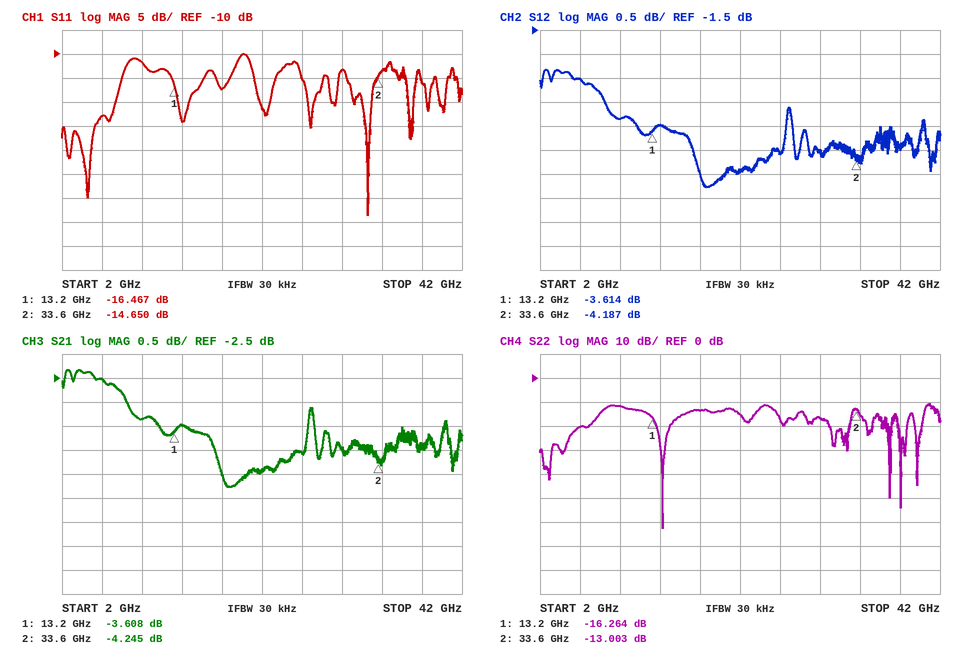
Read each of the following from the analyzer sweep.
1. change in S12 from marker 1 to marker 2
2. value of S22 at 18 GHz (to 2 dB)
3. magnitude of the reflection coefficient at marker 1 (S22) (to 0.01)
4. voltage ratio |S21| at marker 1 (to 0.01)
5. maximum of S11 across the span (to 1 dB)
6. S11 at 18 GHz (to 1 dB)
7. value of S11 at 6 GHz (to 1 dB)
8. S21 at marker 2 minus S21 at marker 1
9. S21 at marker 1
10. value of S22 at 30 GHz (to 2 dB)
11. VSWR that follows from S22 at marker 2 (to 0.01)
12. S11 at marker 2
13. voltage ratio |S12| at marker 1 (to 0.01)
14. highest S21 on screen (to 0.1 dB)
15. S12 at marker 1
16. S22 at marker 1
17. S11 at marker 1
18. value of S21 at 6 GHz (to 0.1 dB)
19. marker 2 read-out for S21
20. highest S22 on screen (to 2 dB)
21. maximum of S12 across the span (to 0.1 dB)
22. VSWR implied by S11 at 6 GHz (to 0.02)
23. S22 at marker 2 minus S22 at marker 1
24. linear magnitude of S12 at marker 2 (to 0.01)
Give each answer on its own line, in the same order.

-0.573 dB
-14 dB
0.15
0.66
-10 dB
-17 dB
-23 dB
-0.637 dB
-3.608 dB
-16 dB
1.58
-14.650 dB
0.66
-2.3 dB
-3.614 dB
-16.264 dB
-16.467 dB
-2.5 dB
-4.245 dB
-10 dB
-2.3 dB
1.16
3.261 dB
0.62
